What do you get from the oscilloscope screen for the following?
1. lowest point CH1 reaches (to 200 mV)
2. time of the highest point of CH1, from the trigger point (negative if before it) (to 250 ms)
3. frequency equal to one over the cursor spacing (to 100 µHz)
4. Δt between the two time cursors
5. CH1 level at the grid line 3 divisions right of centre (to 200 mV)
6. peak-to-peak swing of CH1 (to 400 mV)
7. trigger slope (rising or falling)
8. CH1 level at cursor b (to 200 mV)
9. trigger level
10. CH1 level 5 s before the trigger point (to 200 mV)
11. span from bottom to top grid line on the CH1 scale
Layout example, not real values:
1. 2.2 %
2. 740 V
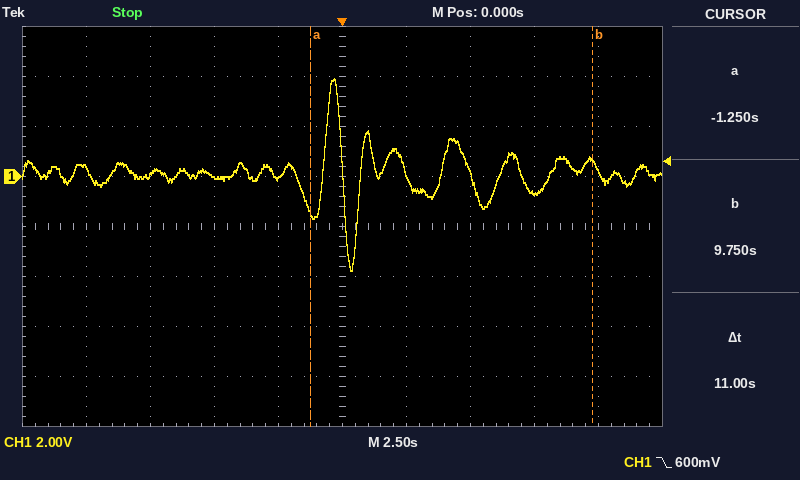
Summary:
1. -3.8 V
2. -250 ms
3. 90.9 mHz
4. 11 s
5. -600 mV
6. 7.6 V
7. falling
8. 600 mV
9. 600 mV
10. 0.0 V
11. 16 V
